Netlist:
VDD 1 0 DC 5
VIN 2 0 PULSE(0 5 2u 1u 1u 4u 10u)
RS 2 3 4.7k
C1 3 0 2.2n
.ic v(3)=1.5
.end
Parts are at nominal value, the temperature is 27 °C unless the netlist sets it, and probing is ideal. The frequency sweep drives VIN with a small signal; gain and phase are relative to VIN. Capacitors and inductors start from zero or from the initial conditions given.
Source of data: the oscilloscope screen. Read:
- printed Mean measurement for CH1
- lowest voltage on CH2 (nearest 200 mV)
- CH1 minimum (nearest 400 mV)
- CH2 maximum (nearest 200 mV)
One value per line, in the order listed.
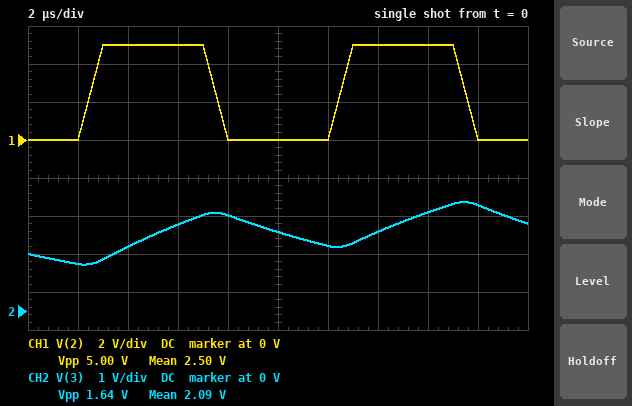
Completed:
2.50 V
1.2 V
0 V
2.8 V
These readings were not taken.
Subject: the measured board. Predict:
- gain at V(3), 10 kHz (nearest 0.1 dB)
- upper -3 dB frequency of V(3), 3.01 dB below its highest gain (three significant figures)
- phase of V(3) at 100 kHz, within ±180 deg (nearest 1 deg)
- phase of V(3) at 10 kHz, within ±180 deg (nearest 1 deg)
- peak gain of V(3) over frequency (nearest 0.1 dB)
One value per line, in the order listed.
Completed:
-1.5 dB
15.4 kHz
-81 deg
-33 deg
0 dB
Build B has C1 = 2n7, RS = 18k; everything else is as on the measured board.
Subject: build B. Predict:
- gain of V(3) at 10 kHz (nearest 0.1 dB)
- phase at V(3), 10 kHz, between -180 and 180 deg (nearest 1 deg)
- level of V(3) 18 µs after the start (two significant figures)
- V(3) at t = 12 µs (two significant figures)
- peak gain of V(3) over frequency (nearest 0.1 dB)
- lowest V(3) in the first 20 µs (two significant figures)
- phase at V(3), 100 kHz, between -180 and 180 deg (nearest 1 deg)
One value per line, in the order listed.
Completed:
-10.1 dB
-72 deg
1.9 V
1.6 V
0 dB
1.4 V
-88 deg
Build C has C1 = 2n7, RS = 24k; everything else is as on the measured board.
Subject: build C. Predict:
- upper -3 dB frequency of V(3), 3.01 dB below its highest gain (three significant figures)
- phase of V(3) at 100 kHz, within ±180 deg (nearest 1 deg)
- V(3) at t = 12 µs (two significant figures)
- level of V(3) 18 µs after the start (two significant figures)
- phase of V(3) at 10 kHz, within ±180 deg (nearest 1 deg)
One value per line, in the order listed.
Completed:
2.46 kHz
-89 deg
1.6 V
1.8 V
-76 deg
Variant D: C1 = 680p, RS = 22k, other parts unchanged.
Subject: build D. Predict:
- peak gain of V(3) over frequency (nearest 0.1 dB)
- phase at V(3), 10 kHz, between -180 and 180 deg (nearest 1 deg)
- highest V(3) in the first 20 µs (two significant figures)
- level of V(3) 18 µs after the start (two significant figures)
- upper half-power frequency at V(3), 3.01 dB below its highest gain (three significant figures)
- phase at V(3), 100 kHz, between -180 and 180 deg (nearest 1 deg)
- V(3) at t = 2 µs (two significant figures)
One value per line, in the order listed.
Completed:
0 dB
-43 deg
2.6 V
2.5 V
10.6 kHz
-84 deg
1.3 V
